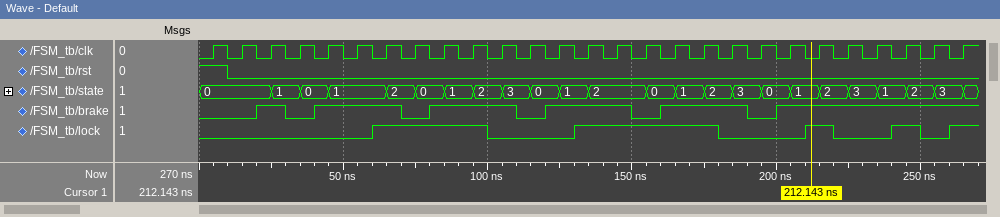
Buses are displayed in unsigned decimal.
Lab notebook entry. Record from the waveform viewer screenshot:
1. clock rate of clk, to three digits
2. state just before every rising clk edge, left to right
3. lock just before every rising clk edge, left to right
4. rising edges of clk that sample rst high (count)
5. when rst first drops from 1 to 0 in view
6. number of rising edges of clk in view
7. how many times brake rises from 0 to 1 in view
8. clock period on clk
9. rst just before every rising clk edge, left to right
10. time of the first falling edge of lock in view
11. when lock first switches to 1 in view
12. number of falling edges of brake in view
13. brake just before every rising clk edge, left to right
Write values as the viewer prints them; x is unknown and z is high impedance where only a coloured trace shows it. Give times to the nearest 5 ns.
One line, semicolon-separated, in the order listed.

100 MHz; 0, 0, 0, 1, 0, 1, 1, 2, 0, 1, 2, 3, 0, 1, 2, 2, 0, 1, 2, 3, 0, 1, 2, 3, 1, 2, 3; 0 0 0 0 0 0 1 1 1 1 0 0 0 1 1 1 1 1 0 0 0 1 0 0 1 0 1; 1; 10 ns; 27; 6; 10 ns; 1 0 0 0 0 0 0 0 0 0 0 0 0 0 0 0 0 0 0 0 0 0 0 0 0 0 0; 100 ns; 60 ns; 5; 0 0 1 0 1 1 1 0 1 1 1 0 1 1 1 0 1 1 1 0 1 1 1 1 1 1 1
